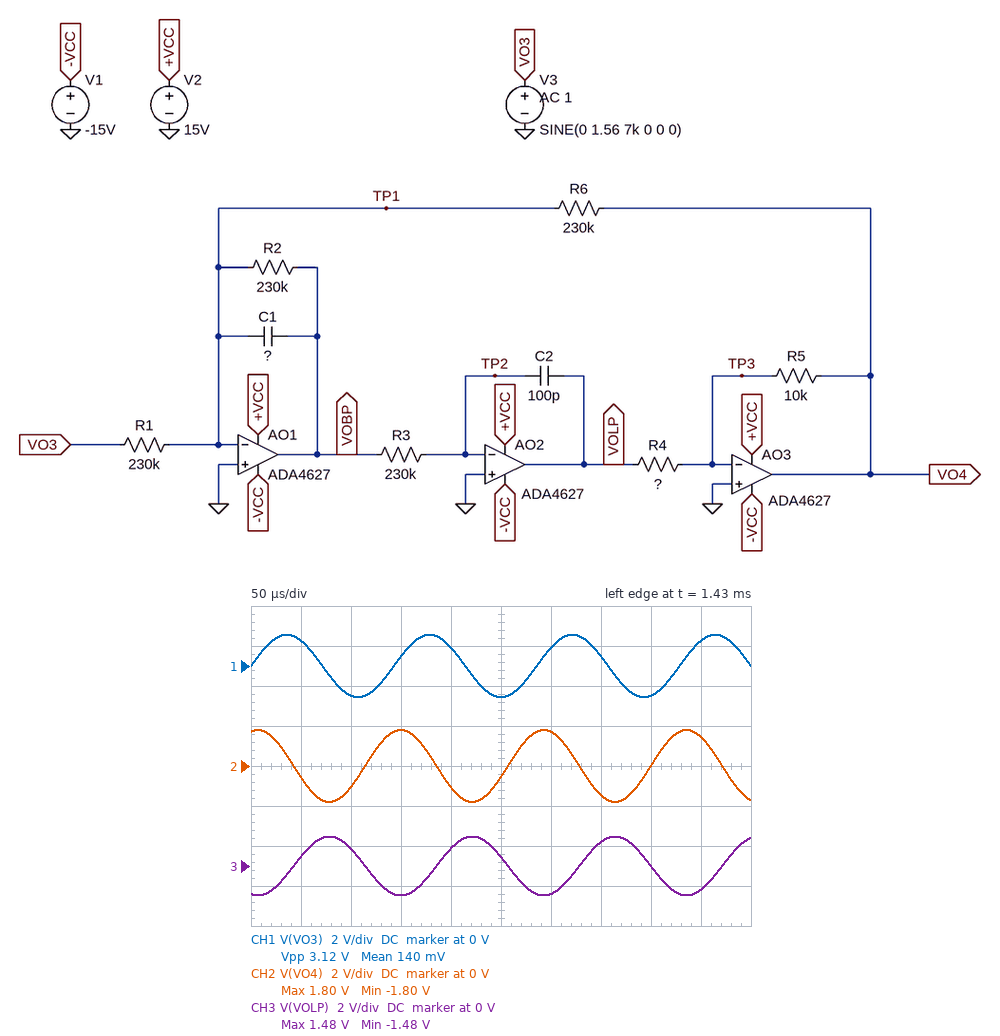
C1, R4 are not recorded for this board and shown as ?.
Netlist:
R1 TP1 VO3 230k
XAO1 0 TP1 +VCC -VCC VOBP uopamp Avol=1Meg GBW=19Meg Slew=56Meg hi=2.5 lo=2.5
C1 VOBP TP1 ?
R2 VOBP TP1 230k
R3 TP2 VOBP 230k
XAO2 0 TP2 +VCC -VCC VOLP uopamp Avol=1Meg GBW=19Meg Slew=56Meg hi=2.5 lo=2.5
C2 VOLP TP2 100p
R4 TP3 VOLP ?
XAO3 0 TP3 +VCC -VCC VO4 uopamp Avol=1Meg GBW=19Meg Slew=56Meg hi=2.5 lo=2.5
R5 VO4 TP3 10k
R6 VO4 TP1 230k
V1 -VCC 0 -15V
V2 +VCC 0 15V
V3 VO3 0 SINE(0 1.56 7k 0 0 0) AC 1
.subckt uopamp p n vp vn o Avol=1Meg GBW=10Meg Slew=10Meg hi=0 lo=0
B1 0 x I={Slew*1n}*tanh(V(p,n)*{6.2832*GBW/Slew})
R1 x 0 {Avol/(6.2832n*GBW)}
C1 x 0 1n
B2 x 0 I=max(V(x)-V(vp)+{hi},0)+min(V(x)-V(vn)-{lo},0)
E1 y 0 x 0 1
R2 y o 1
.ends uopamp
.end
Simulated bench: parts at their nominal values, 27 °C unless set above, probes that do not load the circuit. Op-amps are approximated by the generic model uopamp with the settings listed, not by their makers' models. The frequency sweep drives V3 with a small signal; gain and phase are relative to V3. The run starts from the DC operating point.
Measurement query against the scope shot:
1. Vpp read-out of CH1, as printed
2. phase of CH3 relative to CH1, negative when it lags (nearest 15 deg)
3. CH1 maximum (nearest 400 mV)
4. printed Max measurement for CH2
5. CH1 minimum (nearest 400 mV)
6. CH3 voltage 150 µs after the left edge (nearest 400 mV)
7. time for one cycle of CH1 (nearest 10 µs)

3.12 V
-105 deg
1.6 V
1.80 V
-1.6 V
-1.6 V
140 µs
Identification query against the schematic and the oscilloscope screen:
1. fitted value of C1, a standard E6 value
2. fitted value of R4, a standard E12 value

150 pF
8.2 kΩ
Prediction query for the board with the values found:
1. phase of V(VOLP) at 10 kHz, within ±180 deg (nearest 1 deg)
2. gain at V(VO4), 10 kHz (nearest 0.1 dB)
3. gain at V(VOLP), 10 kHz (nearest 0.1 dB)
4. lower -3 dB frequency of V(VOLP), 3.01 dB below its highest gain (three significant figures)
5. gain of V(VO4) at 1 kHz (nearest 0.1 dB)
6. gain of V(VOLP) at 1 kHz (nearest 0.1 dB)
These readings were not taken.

-143 deg
-5.9 dB
-7.6 dB
1.28 kHz
0.2 dB
-1.6 dB
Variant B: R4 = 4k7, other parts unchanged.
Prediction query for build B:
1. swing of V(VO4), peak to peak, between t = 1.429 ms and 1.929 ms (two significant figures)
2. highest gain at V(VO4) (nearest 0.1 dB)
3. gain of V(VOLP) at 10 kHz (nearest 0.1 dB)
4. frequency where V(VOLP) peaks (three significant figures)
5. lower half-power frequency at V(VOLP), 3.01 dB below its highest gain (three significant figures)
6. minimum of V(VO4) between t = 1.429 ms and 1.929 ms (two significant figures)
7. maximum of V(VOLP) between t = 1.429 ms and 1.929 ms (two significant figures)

5.7 V
5.4 dB
-4.9 dB
7.57 kHz
4.58 kHz
-2.8 V
1.3 V
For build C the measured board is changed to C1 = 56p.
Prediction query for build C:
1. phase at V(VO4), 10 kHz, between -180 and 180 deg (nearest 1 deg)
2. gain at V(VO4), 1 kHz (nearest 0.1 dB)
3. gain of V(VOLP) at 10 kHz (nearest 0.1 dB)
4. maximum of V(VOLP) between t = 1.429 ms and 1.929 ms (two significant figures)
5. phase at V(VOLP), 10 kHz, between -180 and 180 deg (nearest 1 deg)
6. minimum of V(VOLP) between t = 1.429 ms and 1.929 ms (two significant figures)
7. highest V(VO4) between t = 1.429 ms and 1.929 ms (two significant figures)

92 deg
0 dB
-3.2 dB
1.3 V
-88 deg
-1.3 V
1.6 V
